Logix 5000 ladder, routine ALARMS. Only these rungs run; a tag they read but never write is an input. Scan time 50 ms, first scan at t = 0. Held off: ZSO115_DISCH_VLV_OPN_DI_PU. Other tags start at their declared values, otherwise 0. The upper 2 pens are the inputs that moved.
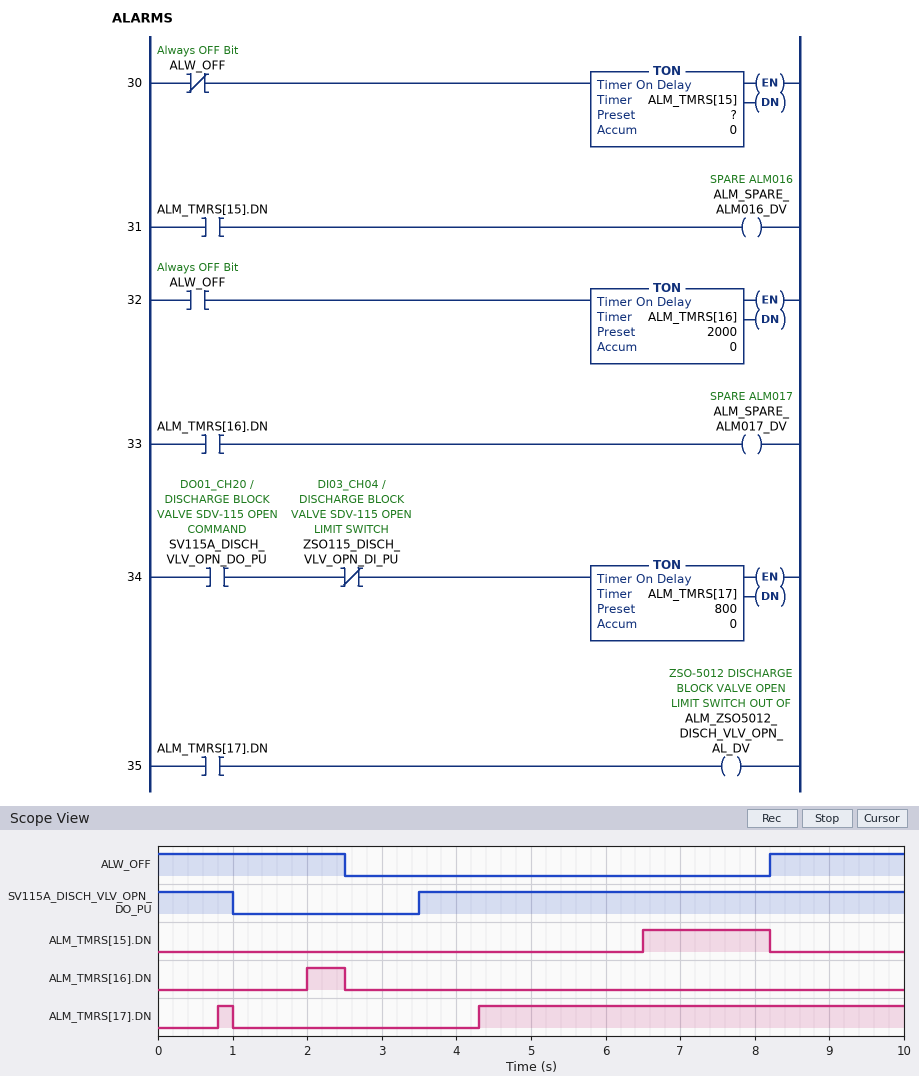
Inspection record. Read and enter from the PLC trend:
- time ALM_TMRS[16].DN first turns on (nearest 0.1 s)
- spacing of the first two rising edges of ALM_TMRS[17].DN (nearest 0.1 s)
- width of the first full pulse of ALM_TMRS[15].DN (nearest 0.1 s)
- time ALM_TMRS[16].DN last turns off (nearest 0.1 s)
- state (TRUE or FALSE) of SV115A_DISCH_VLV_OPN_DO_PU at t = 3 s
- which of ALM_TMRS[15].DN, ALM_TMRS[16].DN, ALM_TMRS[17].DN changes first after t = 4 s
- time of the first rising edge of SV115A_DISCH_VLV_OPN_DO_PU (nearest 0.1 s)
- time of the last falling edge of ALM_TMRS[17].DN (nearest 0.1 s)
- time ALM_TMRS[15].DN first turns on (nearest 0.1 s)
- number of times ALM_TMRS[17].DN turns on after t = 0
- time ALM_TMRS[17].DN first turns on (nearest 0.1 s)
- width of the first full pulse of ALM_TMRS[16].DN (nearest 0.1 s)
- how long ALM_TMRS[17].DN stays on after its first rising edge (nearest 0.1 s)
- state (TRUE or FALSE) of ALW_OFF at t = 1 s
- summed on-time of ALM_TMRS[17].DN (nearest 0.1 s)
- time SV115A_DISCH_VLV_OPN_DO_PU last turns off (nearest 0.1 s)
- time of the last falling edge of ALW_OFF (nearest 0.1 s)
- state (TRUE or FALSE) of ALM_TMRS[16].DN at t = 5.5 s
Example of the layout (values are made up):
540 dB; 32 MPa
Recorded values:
2.0 s; 3.5 s; 1.7 s; 2.5 s; FALSE; ALM_TMRS[17].DN; 3.5 s; 1.0 s; 6.5 s; 2; 0.8 s; 0.5 s; 0.2 s; TRUE; 5.9 s; 1.0 s; 2.5 s; FALSE
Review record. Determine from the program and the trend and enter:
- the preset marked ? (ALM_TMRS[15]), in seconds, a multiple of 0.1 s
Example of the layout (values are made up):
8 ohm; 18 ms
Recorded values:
4.0 s
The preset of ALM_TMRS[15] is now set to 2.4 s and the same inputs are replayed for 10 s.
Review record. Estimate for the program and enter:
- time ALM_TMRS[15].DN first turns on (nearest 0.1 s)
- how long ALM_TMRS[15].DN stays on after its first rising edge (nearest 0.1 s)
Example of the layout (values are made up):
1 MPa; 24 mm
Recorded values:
4.9 s; 3.3 s
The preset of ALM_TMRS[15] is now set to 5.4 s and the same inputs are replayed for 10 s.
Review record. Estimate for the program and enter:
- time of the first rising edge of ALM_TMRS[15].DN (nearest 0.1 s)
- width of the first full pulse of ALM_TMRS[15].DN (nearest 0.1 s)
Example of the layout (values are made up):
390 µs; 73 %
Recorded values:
7.9 s; 0.3 s
